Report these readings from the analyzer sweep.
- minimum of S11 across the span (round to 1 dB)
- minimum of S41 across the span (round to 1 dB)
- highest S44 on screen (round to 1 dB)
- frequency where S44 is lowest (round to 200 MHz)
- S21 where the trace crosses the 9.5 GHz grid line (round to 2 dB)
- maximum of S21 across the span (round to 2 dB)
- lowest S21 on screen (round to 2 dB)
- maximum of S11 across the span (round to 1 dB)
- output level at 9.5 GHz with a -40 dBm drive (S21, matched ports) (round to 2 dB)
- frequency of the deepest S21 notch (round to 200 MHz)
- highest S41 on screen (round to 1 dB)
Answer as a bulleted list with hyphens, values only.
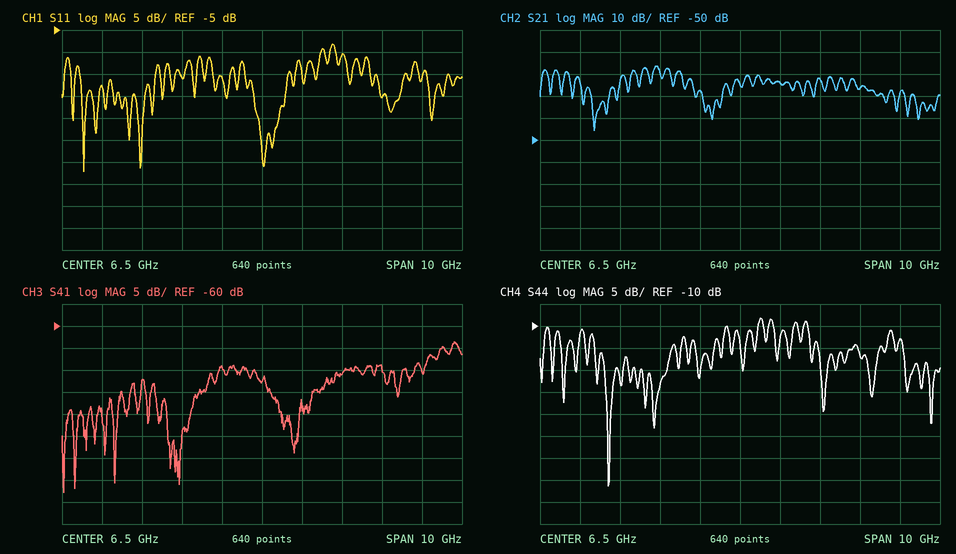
- -37 dB
- -98 dB
- -8 dB
- 3.2 GHz
- -26 dB
- -16 dB
- -46 dB
- -8 dB
- -66 dBm
- 2.8 GHz
- -64 dB
